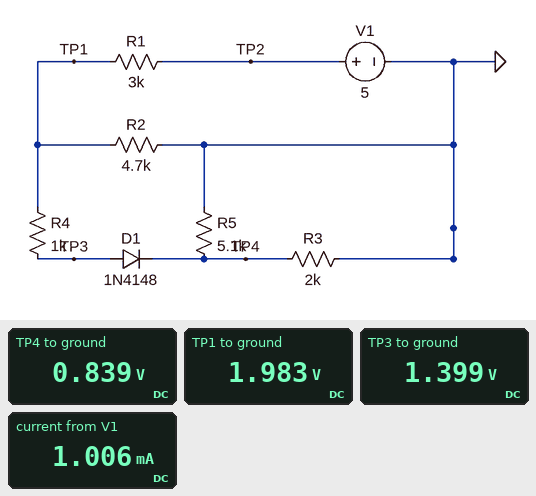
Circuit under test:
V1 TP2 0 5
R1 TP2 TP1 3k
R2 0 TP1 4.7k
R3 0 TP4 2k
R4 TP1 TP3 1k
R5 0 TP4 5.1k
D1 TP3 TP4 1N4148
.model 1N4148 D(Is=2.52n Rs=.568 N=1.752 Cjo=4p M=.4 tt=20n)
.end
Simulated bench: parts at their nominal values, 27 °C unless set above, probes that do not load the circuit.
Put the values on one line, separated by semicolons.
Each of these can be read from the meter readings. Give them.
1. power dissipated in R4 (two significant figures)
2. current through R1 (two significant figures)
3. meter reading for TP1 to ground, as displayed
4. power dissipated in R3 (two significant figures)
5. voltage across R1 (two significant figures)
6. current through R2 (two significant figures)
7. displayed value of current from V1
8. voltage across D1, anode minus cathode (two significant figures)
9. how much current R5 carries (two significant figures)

340 µW; 1.0 mA; 1.983 V; 350 µW; 3.0 V; 420 µA; 1.006 mA; 560 mV; 160 µA
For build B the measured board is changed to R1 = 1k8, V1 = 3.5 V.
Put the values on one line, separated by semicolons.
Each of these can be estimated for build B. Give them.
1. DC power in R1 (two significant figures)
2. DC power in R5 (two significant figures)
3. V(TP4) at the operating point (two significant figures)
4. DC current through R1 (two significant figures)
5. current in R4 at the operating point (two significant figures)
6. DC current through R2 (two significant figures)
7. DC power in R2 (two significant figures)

1.5 mW; 110 µW; 760 mV; 920 µA; 530 µA; 390 µA; 720 µW
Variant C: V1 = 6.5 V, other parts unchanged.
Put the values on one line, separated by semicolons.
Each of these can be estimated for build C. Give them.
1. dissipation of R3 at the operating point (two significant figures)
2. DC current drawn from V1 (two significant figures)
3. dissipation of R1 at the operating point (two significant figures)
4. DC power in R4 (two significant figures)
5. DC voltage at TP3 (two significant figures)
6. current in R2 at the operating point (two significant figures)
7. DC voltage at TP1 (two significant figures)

650 µW; 1.3 mA; 5.3 mW; 630 µW; 1.7 V; 530 µA; 2.5 V
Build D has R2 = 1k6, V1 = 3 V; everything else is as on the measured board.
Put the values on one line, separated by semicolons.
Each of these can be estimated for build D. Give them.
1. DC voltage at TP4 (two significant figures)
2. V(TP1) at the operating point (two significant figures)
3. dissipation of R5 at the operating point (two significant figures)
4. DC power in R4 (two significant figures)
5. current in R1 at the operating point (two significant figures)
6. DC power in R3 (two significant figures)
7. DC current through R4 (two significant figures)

220 mV; 880 mV; 9.9 µW; 24 µW; 710 µA; 25 µW; 160 µA
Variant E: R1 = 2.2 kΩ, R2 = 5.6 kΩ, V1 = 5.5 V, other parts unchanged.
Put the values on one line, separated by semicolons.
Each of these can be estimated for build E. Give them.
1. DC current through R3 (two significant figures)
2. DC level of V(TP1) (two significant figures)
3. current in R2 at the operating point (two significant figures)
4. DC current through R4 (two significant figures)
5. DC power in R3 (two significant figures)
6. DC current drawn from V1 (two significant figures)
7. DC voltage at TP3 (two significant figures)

600 µA; 2.6 V; 470 µA; 840 µA; 730 µW; 1.3 mA; 1.8 V
